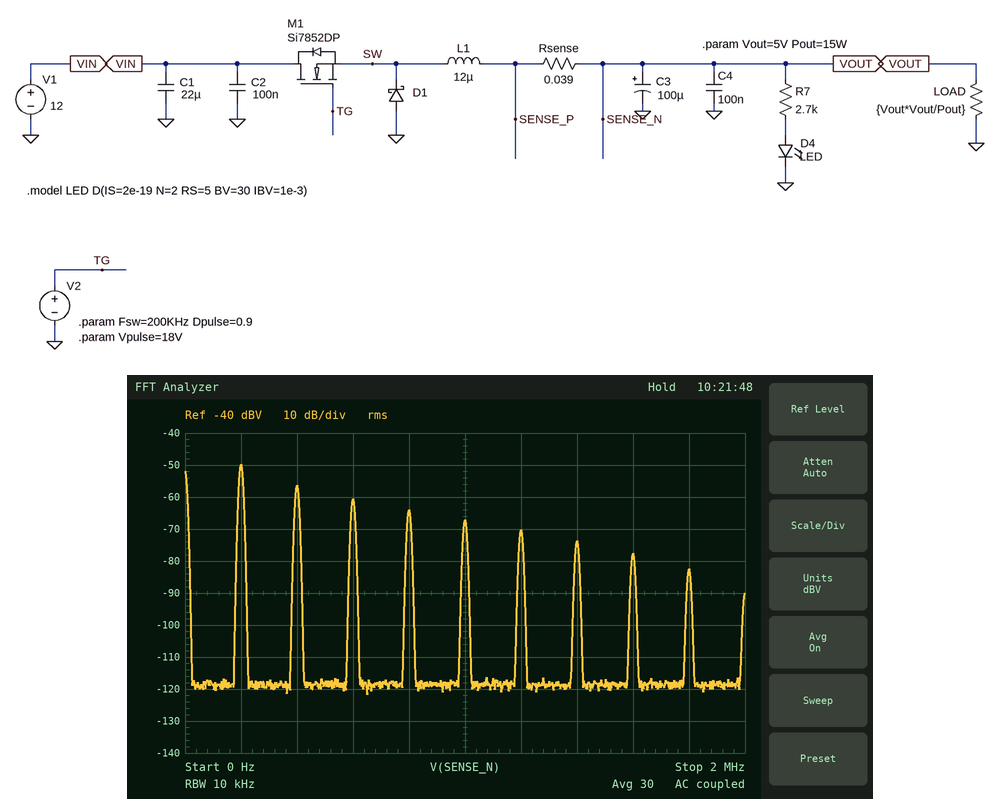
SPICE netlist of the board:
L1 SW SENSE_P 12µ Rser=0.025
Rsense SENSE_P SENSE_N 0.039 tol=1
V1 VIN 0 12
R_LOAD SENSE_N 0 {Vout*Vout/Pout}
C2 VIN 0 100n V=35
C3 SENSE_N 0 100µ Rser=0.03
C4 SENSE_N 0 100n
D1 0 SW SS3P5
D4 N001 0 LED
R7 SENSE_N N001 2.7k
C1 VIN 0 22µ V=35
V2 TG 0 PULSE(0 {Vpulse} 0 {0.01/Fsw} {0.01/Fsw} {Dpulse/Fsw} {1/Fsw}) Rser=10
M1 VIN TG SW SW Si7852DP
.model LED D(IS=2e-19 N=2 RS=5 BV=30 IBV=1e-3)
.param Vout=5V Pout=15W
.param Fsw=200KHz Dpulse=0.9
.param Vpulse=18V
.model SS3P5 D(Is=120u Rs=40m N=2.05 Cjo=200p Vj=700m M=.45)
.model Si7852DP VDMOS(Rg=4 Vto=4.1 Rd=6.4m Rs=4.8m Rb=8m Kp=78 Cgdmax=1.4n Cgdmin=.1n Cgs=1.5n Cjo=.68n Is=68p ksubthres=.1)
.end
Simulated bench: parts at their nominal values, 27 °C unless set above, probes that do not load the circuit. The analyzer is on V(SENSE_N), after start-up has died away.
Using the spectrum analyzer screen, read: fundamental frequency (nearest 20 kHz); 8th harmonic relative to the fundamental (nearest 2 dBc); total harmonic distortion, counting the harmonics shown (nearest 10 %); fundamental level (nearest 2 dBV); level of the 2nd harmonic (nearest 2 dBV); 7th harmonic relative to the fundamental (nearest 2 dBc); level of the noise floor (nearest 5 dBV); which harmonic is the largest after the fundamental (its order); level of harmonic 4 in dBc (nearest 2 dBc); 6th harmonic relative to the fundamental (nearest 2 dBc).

200 kHz
-28 dBc
60 %
-50 dBV
-56 dBV
-24 dBc
-120 dBV
2
-14 dBc
-20 dBc
